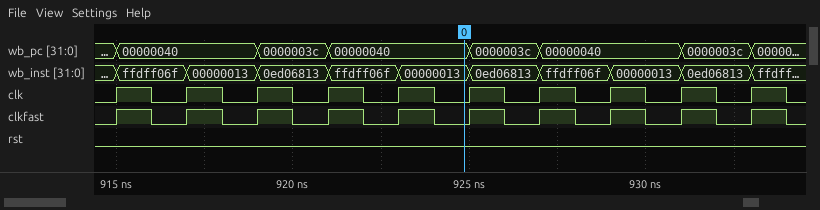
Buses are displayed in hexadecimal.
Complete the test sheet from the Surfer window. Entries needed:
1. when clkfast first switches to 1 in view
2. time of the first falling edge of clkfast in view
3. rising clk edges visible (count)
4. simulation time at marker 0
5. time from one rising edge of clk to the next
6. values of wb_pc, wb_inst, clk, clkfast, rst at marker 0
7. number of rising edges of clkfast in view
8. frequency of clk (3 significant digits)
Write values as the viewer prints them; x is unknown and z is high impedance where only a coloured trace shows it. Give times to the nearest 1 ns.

915 ns
916 ns
10
925 ns
2 ns
wb_pc=00000040, wb_inst=00000013, clk=0, clkfast=0, rst=0
10
500 MHz
